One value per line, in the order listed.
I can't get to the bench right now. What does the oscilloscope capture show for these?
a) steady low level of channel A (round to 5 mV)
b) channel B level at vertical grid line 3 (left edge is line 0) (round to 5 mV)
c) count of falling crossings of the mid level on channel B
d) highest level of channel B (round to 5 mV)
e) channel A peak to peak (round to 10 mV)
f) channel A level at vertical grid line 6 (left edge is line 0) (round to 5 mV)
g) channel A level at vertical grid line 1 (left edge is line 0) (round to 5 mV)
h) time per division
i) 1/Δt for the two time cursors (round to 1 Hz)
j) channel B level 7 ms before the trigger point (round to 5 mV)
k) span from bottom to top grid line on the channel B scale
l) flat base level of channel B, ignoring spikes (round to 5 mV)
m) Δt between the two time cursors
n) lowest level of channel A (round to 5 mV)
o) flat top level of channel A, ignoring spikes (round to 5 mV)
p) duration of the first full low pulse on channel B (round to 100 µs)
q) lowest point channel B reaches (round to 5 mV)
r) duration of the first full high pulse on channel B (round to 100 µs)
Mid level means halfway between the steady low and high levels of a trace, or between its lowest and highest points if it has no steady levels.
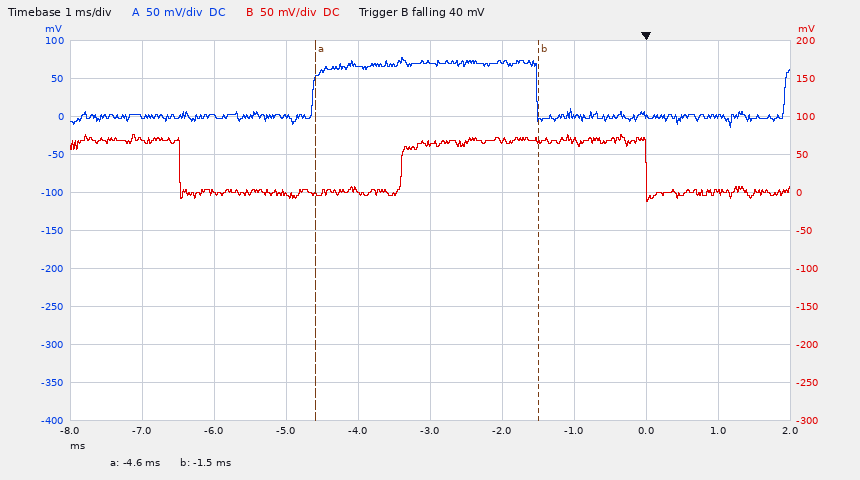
0 mV
0 mV
2
75 mV
90 mV
70 mV
0 mV
1 ms
323 Hz
70 mV
500 mV
0 mV
3.1 ms
-15 mV
70 mV
3.1 ms
-10 mV
3.4 ms
